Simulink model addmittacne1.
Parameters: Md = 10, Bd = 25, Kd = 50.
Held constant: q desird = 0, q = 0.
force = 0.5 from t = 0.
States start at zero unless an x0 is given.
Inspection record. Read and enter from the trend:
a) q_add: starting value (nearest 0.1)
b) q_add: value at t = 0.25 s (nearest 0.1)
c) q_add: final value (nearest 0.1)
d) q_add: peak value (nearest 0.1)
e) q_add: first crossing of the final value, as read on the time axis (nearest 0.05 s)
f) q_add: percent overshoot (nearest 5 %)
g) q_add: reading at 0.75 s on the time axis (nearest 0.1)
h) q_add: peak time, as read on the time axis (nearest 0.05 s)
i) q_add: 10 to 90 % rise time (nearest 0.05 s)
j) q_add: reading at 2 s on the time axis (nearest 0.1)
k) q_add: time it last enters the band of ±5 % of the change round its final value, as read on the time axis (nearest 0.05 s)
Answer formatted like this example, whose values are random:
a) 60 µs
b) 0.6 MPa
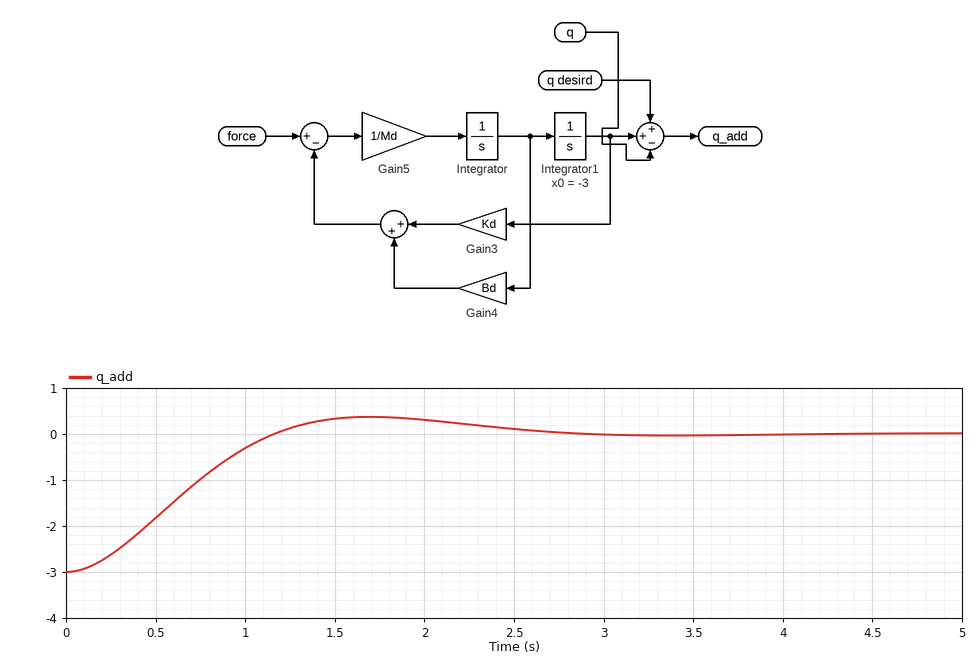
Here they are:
a) -3.0
b) -2.6
c) 0.0
d) 0.4
e) 1.15 s
f) 10 %
g) -1.0
h) 1.70 s
i) 0.80 s
j) 0.3
k) 2.35 s
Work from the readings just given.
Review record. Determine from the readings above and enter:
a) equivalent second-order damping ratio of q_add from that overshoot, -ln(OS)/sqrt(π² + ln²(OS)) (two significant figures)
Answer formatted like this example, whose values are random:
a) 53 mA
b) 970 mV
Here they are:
a) 0.59
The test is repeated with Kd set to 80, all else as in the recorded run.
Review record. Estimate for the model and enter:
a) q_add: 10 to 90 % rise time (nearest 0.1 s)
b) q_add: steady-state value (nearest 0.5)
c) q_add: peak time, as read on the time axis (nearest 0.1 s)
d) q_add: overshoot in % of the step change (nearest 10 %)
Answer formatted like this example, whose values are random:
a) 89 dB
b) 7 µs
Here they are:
a) 0.5 s
b) 0.0
c) 1.2 s
d) 20 %
